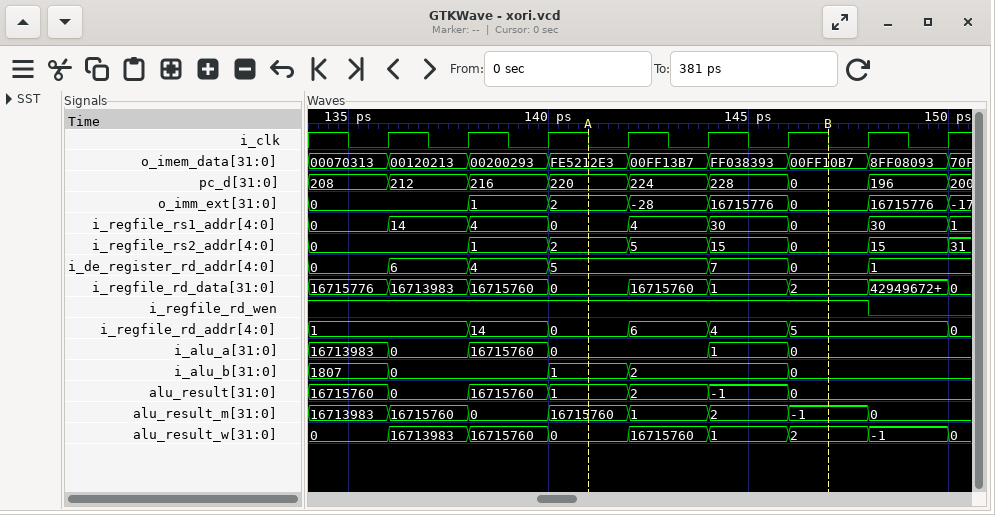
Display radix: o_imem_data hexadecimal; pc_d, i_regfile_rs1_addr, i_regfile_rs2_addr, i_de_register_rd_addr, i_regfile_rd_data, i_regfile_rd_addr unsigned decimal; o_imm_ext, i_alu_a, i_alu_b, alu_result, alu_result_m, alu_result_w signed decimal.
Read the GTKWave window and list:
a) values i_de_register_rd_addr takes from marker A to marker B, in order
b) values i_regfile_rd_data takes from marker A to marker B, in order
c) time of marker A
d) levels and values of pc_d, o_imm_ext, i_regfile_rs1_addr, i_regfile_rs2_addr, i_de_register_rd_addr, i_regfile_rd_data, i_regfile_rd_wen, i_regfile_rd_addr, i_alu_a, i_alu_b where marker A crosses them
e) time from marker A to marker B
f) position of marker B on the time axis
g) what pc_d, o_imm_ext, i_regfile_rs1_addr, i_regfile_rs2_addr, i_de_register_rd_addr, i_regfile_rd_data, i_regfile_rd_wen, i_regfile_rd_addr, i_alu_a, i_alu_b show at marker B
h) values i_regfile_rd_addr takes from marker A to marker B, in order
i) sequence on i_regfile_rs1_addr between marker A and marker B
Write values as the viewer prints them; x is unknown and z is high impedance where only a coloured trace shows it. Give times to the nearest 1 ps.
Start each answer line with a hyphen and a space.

- 5, 7, 0
- 0, 16715760, 1, 2
- 141 ps
- pc_d=220, o_imm_ext=2, i_regfile_rs1_addr=0, i_regfile_rs2_addr=2, i_de_register_rd_addr=5, i_regfile_rd_data=0, i_regfile_rd_wen=1, i_regfile_rd_addr=0, i_alu_a=0, i_alu_b=1
- 6 ps
- 147 ps
- pc_d=0, o_imm_ext=0, i_regfile_rs1_addr=0, i_regfile_rs2_addr=0, i_de_register_rd_addr=0, i_regfile_rd_data=2, i_regfile_rd_wen=1, i_regfile_rd_addr=5, i_alu_a=0, i_alu_b=0
- 0, 6, 4, 5
- 0, 4, 30, 0
